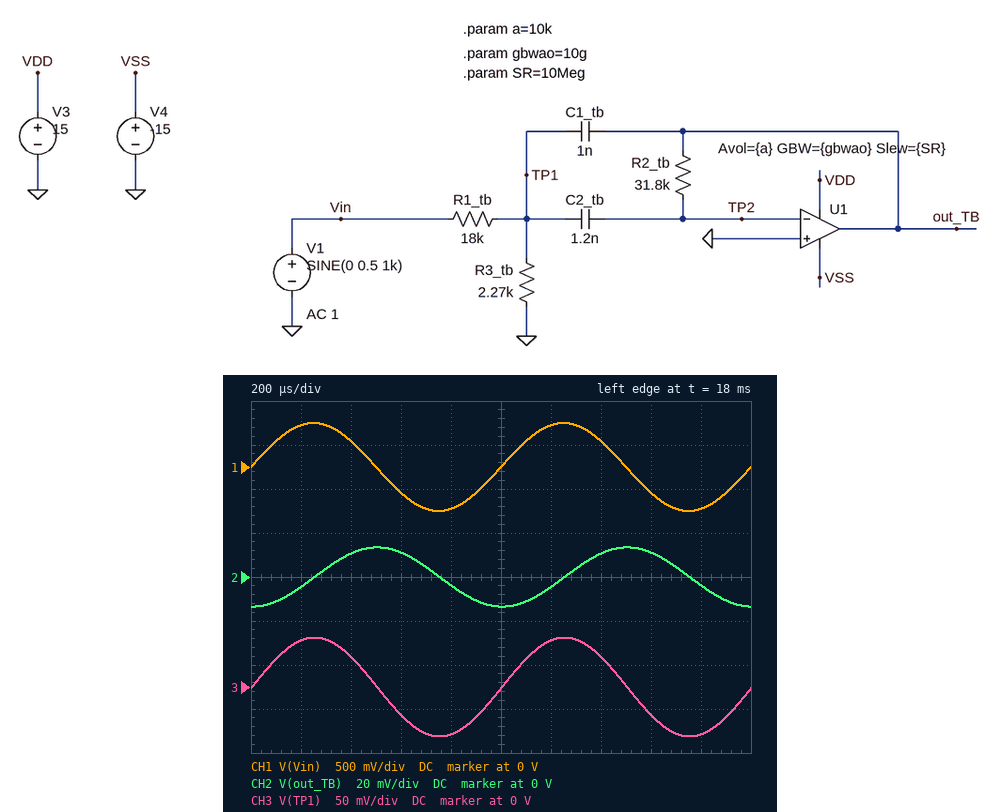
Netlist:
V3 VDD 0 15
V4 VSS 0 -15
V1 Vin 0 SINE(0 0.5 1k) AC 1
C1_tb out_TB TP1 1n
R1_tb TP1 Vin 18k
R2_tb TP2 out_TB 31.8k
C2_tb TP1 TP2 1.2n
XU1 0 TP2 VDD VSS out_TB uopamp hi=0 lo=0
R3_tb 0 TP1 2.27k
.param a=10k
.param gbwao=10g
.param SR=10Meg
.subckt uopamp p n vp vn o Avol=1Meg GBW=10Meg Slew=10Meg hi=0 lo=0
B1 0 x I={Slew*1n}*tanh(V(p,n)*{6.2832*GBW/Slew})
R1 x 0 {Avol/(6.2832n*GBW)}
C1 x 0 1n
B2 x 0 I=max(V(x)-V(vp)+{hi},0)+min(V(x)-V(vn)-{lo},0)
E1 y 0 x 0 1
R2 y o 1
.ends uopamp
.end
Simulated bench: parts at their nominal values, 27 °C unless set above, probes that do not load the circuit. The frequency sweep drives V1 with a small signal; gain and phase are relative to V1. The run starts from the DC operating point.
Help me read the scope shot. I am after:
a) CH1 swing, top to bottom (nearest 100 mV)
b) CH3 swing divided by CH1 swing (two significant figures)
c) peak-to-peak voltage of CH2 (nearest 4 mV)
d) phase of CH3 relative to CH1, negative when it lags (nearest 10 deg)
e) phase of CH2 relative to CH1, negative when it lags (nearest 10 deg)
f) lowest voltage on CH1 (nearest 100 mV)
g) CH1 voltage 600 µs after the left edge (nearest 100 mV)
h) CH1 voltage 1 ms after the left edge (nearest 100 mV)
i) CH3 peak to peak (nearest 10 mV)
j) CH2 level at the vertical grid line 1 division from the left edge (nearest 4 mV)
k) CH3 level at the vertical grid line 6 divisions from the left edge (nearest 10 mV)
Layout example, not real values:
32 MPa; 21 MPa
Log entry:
1.0 V; 0.11; 28 mV; 0 deg; -90 deg; -500 mV; -300 mV; 0 V; 110 mV; -4 mV; 50 mV
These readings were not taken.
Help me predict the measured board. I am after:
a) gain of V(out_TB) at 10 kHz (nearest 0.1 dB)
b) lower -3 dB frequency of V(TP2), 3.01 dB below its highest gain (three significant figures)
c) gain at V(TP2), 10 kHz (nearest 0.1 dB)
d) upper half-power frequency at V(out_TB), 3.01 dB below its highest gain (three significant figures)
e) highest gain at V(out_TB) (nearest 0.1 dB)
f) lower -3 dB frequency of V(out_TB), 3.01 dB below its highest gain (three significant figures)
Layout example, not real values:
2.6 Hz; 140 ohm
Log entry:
-8.9 dB; 15.5 kHz; -68.9 dB; 23.2 kHz; -0.3 dB; 14.1 kHz
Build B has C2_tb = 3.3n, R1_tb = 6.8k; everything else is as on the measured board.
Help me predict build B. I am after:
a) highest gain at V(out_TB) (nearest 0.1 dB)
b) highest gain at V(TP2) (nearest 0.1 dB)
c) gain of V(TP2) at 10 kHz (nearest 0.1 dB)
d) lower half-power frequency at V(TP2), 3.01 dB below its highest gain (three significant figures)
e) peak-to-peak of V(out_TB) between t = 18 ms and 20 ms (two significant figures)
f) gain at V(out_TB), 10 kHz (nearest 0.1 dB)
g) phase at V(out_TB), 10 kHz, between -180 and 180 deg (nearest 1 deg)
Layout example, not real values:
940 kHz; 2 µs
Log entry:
11.1 dB; -47.1 dB; -50.3 dB; 10.1 kHz; 170 mV; 9.7 dB; -148 deg
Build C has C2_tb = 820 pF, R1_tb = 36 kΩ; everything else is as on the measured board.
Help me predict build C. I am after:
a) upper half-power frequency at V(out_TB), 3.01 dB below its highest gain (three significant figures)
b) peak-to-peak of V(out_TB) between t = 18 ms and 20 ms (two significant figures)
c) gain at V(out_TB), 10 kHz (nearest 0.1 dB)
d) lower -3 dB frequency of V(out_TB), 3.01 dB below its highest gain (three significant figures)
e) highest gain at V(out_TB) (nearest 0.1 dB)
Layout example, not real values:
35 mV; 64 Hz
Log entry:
27.5 kHz; 9.7 mV; -18.5 dB; 16.4 kHz; -8.0 dB
